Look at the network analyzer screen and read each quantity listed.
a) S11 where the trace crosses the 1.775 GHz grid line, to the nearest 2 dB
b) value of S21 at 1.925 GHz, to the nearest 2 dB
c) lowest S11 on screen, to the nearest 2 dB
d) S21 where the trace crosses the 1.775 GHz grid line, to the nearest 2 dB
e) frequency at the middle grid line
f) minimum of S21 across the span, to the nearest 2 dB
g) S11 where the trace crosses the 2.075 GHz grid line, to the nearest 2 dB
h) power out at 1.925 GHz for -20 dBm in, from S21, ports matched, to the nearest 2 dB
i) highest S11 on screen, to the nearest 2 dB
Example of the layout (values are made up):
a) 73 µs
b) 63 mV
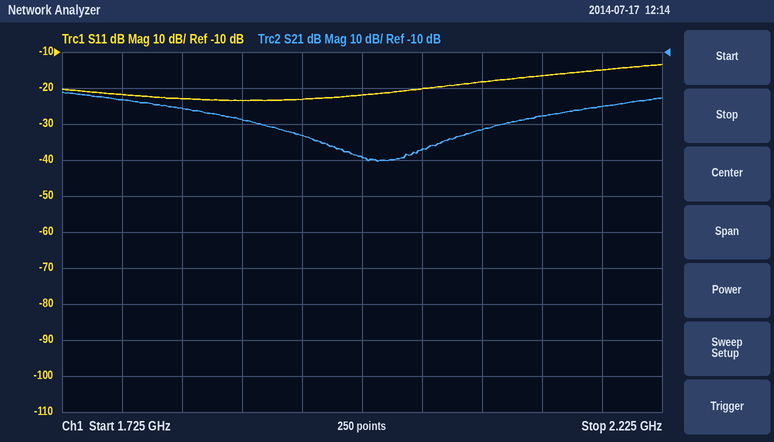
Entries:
a) -22 dB
b) -34 dB
c) -24 dB
d) -24 dB
e) 1.975 GHz
f) -40 dB
g) -18 dB
h) -54 dBm
i) -14 dB
